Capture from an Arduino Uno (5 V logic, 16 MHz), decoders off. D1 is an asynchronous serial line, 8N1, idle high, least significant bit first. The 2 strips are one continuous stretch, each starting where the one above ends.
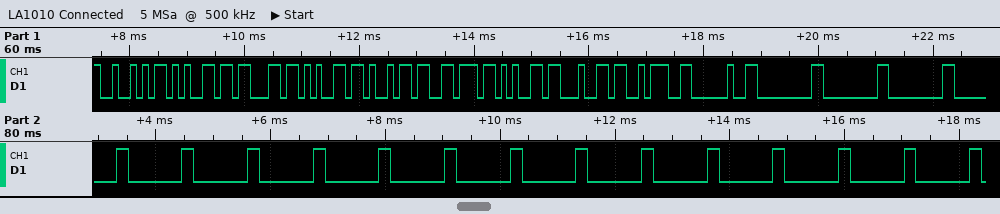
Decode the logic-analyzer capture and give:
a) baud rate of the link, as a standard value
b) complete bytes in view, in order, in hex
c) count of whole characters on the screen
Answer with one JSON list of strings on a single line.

["9600 baud", "0x52 0x65 0x63 0x65 0x69 0x76 0x65 0x64 0x3A 0x20 0x00 0x00 0x00 0x00 0x00 0x00 0x00 0x00 0x00 0x00 0x00 0x00 0x00 0x00 0x00 0x00 0x00", "27"]
